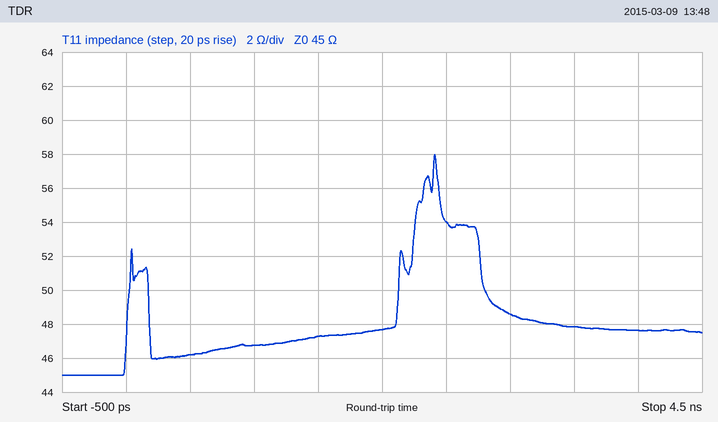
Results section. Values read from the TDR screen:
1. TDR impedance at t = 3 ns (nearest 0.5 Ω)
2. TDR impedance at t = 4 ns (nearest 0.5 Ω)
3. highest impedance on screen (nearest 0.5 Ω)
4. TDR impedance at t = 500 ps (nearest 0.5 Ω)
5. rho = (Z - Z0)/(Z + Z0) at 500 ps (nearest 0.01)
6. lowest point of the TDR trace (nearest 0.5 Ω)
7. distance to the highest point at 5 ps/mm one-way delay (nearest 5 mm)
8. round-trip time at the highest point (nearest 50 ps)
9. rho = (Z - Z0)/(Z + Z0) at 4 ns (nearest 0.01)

48.5 Ω
47.5 Ω
58.0 Ω
46.0 Ω
+0.01
45.0 Ω
240 mm
2.40 ns
+0.03
